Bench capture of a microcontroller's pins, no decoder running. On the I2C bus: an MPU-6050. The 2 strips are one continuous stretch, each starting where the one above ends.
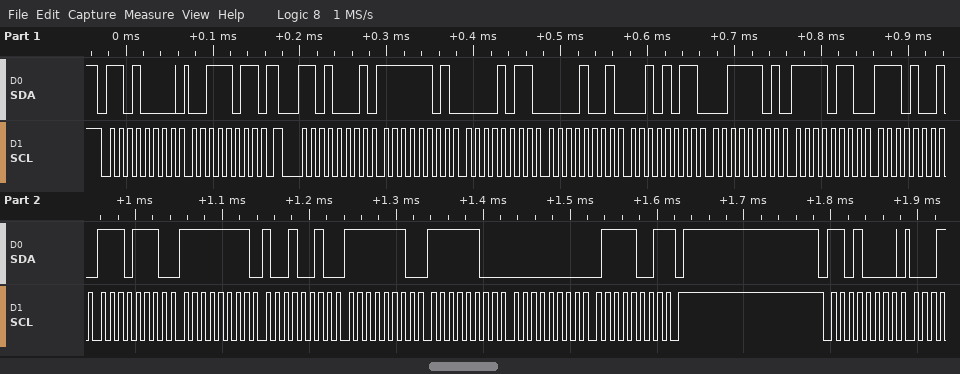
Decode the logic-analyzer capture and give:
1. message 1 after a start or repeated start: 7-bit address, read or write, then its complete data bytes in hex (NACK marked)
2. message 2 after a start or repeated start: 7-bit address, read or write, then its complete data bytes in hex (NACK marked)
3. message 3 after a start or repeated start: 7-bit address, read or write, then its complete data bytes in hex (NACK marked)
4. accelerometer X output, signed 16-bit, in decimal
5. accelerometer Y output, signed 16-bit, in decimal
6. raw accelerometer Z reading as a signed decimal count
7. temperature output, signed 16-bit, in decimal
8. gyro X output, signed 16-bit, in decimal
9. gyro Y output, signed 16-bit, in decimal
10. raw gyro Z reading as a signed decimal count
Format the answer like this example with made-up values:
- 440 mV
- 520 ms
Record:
- 0x68 write: 3B
- 0x68 read: FD 0B 09 2B 3D F6 E9 EE FF 92 FE FC 00 79 NACK
- 0x68 write
- -757
- 2347
- 15862
- -5650
- -110
- -260
- 121
